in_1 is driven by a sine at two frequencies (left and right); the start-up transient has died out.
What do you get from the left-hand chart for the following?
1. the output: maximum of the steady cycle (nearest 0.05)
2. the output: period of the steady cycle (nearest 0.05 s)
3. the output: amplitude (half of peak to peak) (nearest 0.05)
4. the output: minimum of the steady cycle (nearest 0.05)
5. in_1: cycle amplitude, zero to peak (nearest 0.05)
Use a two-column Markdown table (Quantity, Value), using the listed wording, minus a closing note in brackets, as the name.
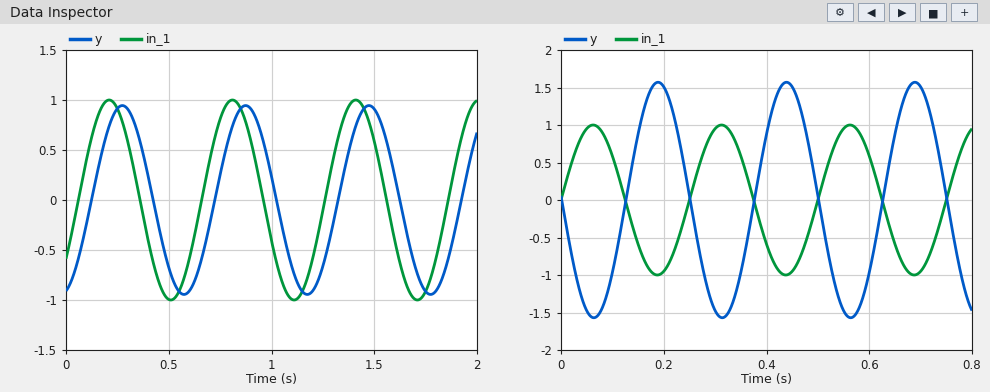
| Quantity | Value |
|---|---|
| the output: maximum of the steady cycle | 0.95 |
| the output: period of the steady cycle | 0.60 s |
| the output: amplitude (half of peak to peak) | 0.95 |
| the output: minimum of the steady cycle | -0.95 |
| in_1: cycle amplitude, zero to peak | 1.00 |
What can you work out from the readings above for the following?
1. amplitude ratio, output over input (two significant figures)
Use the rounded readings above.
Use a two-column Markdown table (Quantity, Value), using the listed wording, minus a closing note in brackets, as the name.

| Quantity | Value |
|---|---|
| amplitude ratio, output over input | 0.95 |
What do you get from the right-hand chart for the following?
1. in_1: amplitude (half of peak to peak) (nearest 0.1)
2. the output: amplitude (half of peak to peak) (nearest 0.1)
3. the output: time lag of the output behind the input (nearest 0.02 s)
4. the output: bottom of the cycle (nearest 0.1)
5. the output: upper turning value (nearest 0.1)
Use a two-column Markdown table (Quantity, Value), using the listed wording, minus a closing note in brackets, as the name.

| Quantity | Value |
|---|---|
| in_1: amplitude (half of peak to peak) | 1.0 |
| the output: amplitude (half of peak to peak) | 1.6 |
| the output: time lag of the output behind the input | 0.12 s |
| the output: bottom of the cycle | -1.6 |
| the output: upper turning value | 1.6 |
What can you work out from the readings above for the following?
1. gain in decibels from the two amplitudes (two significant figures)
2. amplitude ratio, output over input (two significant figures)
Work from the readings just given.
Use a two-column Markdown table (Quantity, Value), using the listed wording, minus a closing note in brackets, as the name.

| Quantity | Value |
|---|---|
| gain in decibels from the two amplitudes | 4.1 dB |
| amplitude ratio, output over input | 1.6 |
